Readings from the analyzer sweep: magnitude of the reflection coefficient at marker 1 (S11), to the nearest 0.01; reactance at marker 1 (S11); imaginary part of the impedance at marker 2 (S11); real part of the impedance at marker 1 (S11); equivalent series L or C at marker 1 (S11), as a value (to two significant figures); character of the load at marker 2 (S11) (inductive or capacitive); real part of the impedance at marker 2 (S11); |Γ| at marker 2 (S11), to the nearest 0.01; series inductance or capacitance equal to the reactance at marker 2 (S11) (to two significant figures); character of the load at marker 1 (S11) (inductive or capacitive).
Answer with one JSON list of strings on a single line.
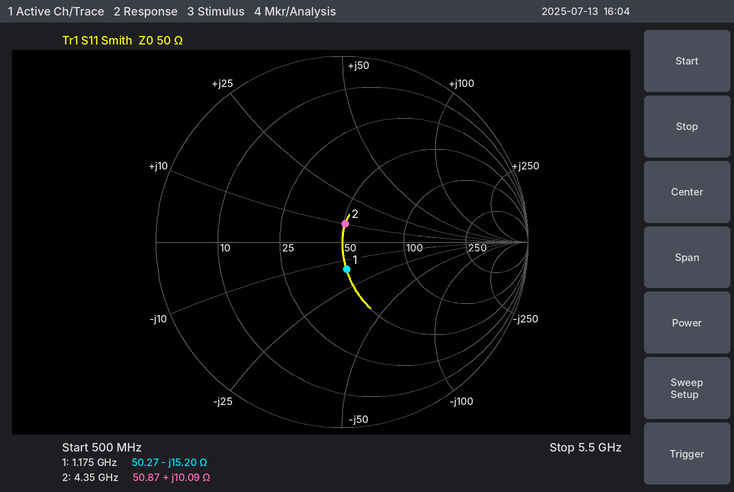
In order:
["0.15", "-15.20 Ω", "+10.09 Ω", "50.27 Ω", "8.9 pF", "inductive", "50.87 Ω", "0.10", "370 pH", "capacitive"]
